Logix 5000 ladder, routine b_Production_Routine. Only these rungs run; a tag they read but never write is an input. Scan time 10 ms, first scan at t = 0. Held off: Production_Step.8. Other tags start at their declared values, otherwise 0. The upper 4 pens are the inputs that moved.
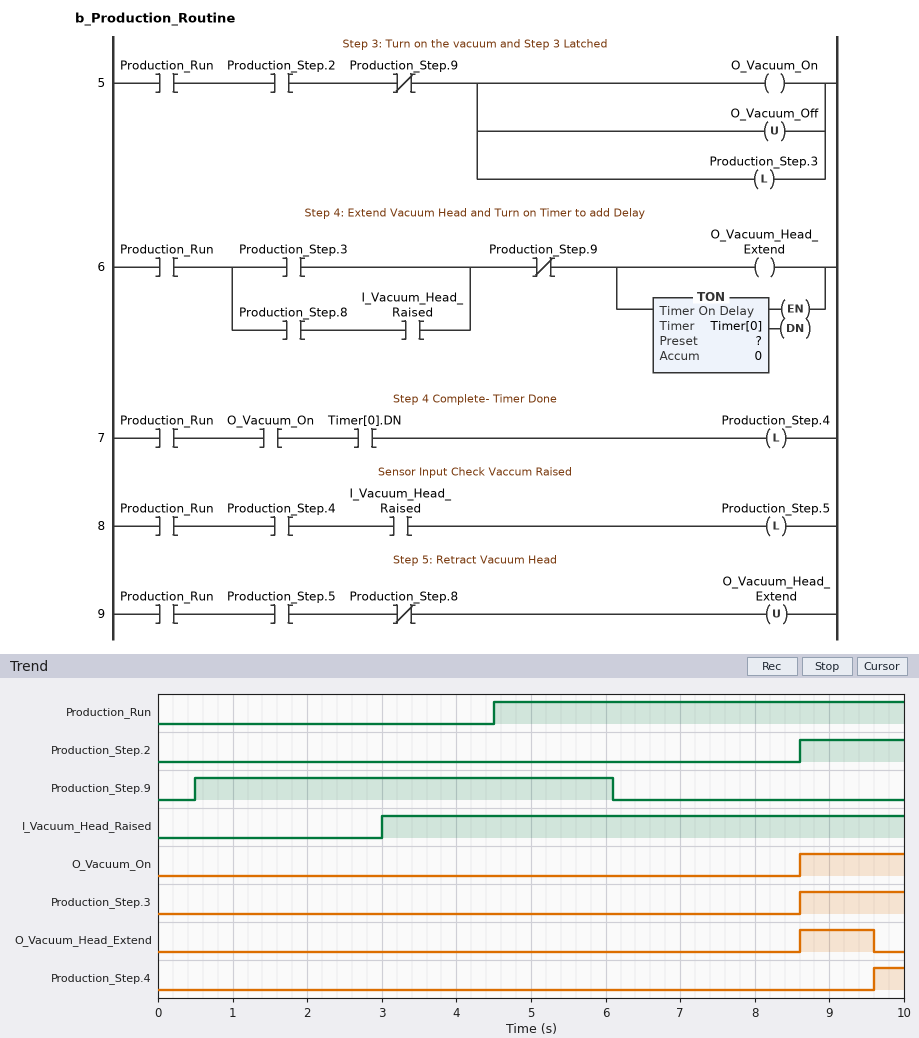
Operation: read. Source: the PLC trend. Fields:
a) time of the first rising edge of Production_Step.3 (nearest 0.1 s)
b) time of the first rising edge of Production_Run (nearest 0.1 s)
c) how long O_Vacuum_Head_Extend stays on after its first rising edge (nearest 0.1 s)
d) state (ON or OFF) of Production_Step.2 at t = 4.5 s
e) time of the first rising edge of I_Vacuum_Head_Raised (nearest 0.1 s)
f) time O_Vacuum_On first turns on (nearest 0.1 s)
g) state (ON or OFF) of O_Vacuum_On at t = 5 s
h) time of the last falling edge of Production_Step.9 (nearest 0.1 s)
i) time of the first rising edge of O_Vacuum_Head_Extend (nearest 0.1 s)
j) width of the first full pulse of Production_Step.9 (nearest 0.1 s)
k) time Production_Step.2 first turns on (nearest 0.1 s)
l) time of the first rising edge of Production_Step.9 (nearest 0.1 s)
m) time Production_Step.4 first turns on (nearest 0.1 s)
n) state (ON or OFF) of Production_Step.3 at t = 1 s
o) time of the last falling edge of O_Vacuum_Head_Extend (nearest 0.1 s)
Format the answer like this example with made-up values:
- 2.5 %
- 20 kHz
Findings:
- 8.6 s
- 4.5 s
- 1.0 s
- OFF
- 3.0 s
- 8.6 s
- OFF
- 6.1 s
- 8.6 s
- 5.6 s
- 8.6 s
- 0.5 s
- 9.6 s
- OFF
- 9.6 s
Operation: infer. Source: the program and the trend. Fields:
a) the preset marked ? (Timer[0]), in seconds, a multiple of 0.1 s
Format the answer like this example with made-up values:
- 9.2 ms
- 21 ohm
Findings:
- 1.0 s
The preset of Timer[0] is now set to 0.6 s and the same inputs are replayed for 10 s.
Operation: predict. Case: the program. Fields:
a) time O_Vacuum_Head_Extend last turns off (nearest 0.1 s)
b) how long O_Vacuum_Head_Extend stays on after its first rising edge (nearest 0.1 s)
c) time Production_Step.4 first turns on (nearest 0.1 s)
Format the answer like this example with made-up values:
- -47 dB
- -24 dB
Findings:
- 9.2 s
- 0.6 s
- 9.2 s
